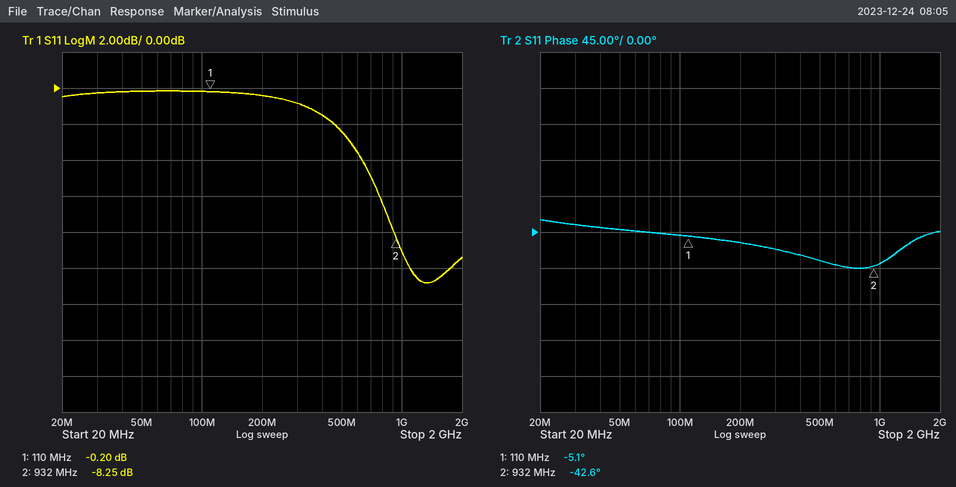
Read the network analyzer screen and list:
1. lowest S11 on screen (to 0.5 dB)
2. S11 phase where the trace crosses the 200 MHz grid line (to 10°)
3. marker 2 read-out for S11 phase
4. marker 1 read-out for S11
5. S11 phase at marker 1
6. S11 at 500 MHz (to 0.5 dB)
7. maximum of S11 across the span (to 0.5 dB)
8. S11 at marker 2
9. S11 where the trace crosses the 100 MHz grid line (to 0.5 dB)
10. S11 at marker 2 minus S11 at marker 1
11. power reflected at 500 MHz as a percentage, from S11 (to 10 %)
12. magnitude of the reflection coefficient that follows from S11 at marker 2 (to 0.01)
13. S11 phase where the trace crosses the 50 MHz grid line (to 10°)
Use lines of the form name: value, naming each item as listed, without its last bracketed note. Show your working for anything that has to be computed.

lowest S11 on screen: -11.0 dB
S11 phase where the trace crosses the 200 MHz grid line: -10°
marker 2 read-out for S11 phase: -42.6°
marker 1 read-out for S11: -0.20 dB
S11 phase at marker 1: -5.1°
S11 at 500 MHz: -2.5 dB
maximum of S11 across the span: 0.0 dB
S11 at marker 2: -8.25 dB
S11 where the trace crosses the 100 MHz grid line: 0.0 dB
S11 at marker 2 minus S11 at marker 1: -8.25 − (-0.2) = -8.05 dB
power reflected at 500 MHz as a percentage, from S11: 10^(-2.5/10) ≈ 56.2 %, so 60 % to the nearest 10 %
magnitude of the reflection coefficient that follows from S11 at marker 2: 10^(-8.25/20) ≈ 0.39
S11 phase where the trace crosses the 50 MHz grid line: 0°
